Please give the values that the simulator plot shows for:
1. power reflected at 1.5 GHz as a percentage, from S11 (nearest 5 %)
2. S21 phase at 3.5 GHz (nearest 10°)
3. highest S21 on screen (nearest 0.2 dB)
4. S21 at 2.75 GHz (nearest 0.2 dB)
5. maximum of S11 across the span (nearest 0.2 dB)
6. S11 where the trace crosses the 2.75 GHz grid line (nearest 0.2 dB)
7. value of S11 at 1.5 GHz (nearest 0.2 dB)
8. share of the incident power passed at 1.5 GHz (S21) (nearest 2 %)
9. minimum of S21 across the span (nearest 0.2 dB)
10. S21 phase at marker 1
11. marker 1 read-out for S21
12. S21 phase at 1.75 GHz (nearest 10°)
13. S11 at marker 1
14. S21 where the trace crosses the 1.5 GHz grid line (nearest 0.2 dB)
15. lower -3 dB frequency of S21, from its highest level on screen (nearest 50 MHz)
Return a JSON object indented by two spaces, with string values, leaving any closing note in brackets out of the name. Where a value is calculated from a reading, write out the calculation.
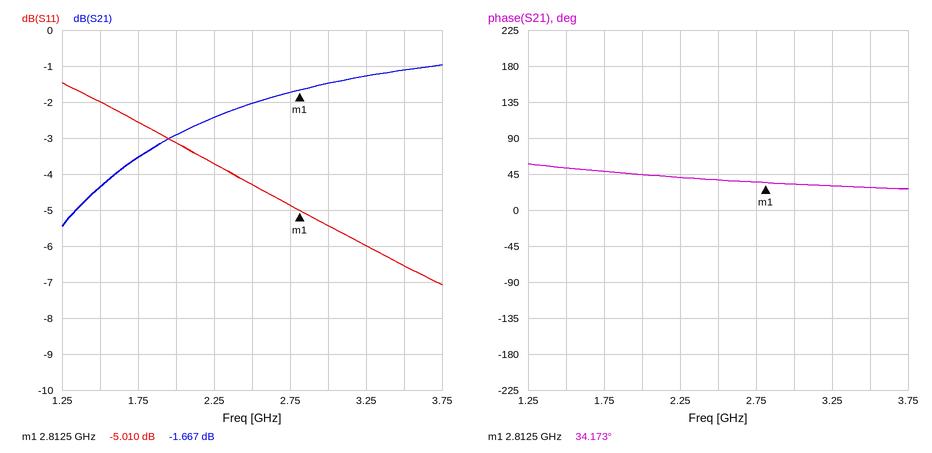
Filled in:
{
  "power reflected at 1.5 GHz as a percentage, from S11": "10^(-2/10) ≈ 63.1 %, so 65 % to the nearest 5 %",
  "S21 phase at 3.5 GHz": "30°",
  "highest S21 on screen": "-1.0 dB",
  "S21 at 2.75 GHz": "-1.8 dB",
  "maximum of S11 across the span": "-1.4 dB",
  "S11 where the trace crosses the 2.75 GHz grid line": "-4.8 dB",
  "value of S11 at 1.5 GHz": "-2.0 dB",
  "share of the incident power passed at 1.5 GHz (S21)": "10^(-4.4/10) ≈ 36 %",
  "minimum of S21 across the span": "-5.4 dB",
  "S21 phase at marker 1": "34.173°",
  "marker 1 read-out for S21": "-1.667 dB",
  "S21 phase at 1.75 GHz": "50°",
  "S11 at marker 1": "-5.010 dB",
  "S21 where the trace crosses the 1.5 GHz grid line": "-4.4 dB",
  "lower -3 dB frequency of S21, from its highest level on screen": "1.60 GHz"
}
